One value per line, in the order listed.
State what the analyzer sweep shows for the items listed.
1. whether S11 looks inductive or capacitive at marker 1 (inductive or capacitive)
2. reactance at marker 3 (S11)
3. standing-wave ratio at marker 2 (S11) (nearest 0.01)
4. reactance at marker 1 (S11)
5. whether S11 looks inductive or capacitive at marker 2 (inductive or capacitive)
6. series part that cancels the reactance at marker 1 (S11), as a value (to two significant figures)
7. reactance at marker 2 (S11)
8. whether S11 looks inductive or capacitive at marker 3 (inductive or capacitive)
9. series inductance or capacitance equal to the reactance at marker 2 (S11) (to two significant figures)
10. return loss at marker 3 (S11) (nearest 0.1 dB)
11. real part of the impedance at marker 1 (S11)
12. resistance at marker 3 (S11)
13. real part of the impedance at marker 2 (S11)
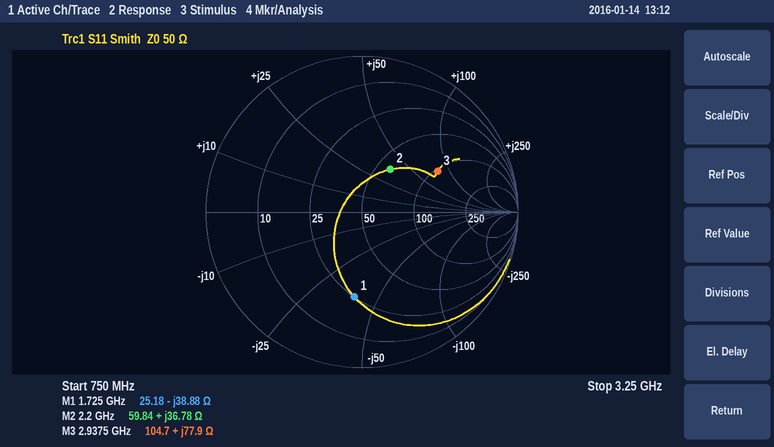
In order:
capacitive
+77.9 Ω
1.98
-38.88 Ω
inductive
3.6 nH
+36.78 Ω
inductive
2.7 nH
5.2 dB
25.18 Ω
104.7 Ω
59.84 Ω
